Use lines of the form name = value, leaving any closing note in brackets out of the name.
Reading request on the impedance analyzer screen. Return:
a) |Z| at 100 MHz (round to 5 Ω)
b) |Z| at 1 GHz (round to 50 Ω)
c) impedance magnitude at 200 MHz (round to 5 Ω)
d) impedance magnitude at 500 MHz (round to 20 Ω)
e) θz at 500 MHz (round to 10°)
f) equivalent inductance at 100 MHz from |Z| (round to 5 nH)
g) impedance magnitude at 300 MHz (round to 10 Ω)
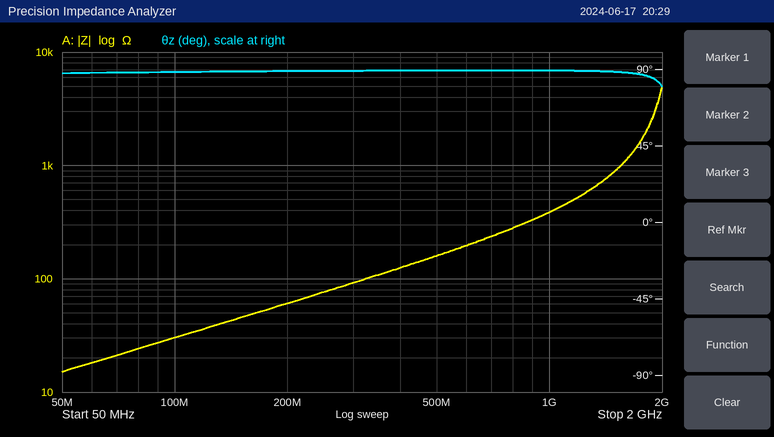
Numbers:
|Z| at 100 MHz = 30 Ω
|Z| at 1 GHz = 400 Ω
impedance magnitude at 200 MHz = 60 Ω
impedance magnitude at 500 MHz = 160 Ω
θz at 500 MHz = 90°
equivalent inductance at 100 MHz from |Z| = 50 nH
impedance magnitude at 300 MHz = 90 Ω
